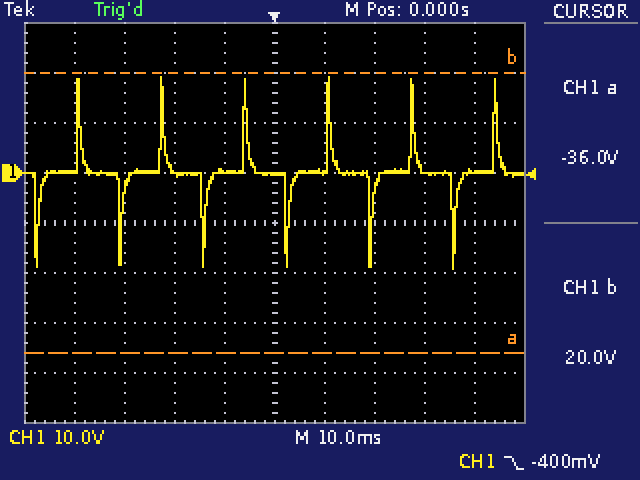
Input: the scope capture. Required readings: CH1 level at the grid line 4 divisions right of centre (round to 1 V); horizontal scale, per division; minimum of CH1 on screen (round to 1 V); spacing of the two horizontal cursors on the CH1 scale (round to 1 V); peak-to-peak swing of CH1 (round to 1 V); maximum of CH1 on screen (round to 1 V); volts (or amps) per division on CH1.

0 V
10 ms
-19 V
56 V
38 V
19 V
10 V
